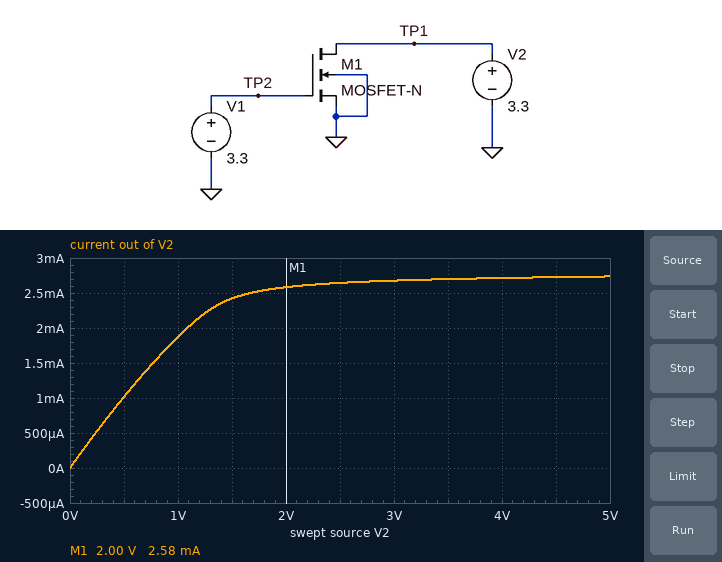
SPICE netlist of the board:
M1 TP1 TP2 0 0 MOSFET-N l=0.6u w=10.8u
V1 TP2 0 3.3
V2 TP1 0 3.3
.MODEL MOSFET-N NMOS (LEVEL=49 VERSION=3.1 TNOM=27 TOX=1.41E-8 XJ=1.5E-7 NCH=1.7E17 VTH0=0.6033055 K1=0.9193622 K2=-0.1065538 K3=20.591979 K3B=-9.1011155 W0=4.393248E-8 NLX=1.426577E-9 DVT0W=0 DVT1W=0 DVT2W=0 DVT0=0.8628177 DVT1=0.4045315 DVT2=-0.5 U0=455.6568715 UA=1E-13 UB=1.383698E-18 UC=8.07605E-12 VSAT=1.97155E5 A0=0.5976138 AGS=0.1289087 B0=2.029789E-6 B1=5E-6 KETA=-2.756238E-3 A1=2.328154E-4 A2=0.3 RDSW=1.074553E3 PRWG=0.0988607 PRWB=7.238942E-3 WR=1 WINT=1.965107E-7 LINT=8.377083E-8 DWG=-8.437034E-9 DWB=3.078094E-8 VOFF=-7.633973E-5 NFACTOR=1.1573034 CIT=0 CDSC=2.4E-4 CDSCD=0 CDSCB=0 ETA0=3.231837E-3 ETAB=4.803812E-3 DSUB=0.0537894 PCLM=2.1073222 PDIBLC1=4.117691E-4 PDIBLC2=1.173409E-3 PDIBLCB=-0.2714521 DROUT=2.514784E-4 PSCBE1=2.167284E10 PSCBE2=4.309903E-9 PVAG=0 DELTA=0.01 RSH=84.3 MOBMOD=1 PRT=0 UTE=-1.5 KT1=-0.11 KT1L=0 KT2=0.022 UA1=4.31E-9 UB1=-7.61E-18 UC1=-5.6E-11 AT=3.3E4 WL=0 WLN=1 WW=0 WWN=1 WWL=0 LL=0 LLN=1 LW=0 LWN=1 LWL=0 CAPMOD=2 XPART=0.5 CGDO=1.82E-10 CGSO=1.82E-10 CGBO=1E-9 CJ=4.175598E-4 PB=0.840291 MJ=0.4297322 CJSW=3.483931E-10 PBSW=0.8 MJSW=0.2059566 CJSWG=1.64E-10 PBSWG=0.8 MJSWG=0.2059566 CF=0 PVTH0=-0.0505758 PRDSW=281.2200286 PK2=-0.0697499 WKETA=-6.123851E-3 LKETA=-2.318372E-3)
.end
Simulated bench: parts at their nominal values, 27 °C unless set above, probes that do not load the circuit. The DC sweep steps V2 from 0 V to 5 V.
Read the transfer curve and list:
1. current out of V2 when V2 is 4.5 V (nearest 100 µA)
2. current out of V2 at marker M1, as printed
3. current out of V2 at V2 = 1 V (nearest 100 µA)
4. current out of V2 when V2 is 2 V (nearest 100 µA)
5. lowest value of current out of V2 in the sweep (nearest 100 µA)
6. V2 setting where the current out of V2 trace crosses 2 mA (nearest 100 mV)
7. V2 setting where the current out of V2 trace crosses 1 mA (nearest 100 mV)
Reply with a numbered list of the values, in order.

1. 2.7 mA
2. 2.58 mA
3. 1.9 mA
4. 2.6 mA
5. 0 A
6. 1.1 V
7. 500 mV
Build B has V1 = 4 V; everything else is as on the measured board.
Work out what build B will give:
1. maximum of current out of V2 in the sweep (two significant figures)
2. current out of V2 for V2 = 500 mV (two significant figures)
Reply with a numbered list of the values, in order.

1. 3.5 mA
2. 1.1 mA
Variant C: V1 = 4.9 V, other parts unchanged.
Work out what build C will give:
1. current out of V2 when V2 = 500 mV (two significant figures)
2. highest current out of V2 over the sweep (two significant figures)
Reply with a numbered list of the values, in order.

1. 1.1 mA
2. 4.5 mA
